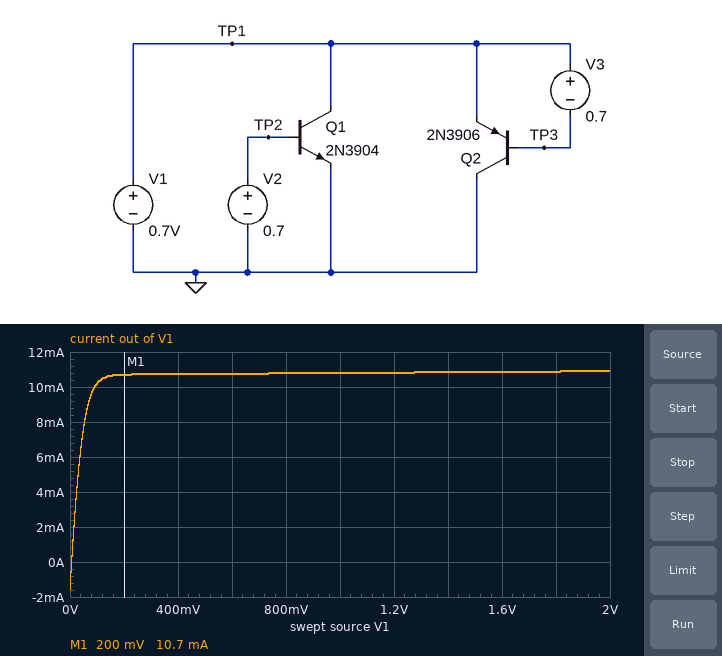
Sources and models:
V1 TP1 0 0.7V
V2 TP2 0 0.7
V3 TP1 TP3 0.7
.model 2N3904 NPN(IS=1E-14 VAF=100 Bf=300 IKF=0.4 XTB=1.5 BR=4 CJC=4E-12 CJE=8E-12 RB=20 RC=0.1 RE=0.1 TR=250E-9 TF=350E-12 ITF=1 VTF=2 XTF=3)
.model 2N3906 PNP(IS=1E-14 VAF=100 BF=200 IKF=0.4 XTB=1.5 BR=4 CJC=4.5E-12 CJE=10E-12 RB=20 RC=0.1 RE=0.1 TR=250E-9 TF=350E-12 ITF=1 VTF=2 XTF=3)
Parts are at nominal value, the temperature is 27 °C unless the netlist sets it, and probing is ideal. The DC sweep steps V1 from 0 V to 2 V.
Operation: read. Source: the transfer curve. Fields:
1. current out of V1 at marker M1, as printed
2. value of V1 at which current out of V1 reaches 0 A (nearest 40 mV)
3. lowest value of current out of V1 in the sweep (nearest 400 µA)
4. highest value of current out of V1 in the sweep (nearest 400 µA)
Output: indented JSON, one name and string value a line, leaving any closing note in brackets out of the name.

{
  "current out of V1 at marker M1, as printed": "10.7 mA",
  "value of V1 at which current out of V1 reaches 0 A": "0 V",
  "lowest value of current out of V1 in the sweep": "-1.6 mA",
  "highest value of current out of V1 in the sweep": "10.8 mA"
}
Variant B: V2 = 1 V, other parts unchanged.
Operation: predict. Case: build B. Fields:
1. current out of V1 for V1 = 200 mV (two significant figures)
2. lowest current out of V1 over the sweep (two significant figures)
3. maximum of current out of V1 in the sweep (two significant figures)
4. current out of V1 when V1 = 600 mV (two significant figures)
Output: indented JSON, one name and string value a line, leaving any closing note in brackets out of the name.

{
  "current out of V1 for V1 = 200 mV": "440 mA",
  "lowest current out of V1 over the sweep": "-11 mA",
  "maximum of current out of V1 in the sweep": "600 mA",
  "current out of V1 when V1 = 600 mV": "590 mA"
}
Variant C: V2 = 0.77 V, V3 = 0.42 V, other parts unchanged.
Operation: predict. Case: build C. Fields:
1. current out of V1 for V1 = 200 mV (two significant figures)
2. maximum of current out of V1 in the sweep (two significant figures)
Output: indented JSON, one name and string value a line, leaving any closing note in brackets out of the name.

{
  "current out of V1 for V1 = 200 mV": "52 mA",
  "maximum of current out of V1 in the sweep": "53 mA"
}
